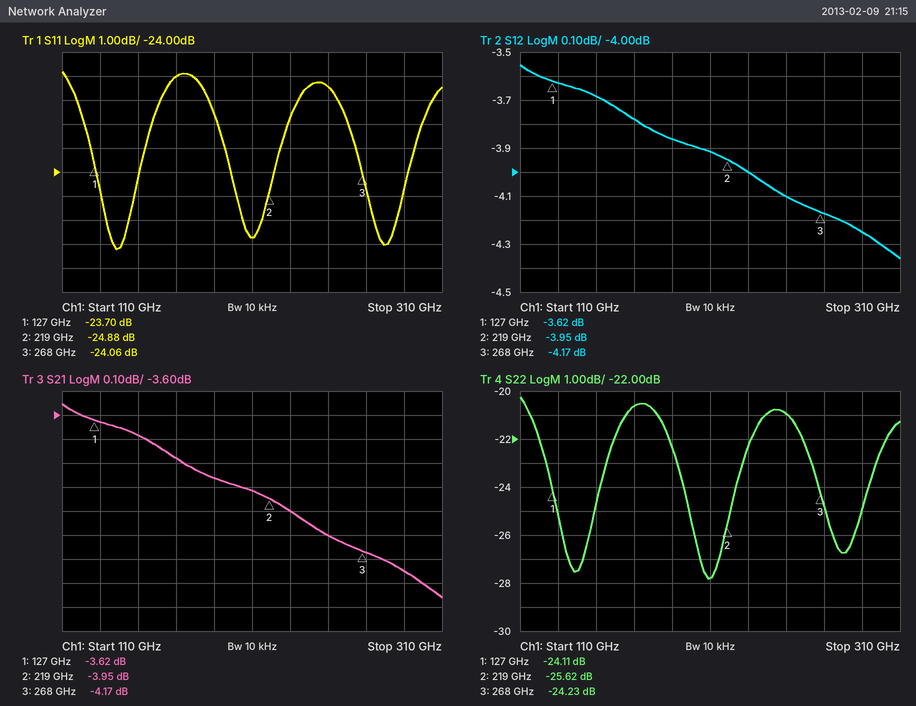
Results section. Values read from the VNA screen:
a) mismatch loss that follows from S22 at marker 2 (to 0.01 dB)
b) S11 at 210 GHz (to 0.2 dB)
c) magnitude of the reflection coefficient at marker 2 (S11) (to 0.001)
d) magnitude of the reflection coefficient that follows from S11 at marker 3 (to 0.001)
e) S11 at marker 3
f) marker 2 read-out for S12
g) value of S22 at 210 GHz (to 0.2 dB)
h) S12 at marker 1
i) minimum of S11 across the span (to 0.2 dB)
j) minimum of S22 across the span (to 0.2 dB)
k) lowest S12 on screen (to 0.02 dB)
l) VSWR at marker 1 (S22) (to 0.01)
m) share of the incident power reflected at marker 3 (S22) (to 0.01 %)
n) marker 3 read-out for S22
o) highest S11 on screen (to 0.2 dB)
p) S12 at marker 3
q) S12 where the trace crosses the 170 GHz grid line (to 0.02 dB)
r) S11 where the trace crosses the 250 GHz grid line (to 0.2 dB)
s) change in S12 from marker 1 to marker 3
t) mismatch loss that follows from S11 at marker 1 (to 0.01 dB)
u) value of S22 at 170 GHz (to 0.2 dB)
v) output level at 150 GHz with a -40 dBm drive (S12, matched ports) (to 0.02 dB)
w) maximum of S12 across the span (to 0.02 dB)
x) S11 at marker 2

0.01 dB
-26.8 dB
0.057
0.063
-24.06 dB
-3.95 dB
-27.8 dB
-3.62 dB
-27.2 dB
-27.8 dB
-4.36 dB
1.13
0.38 %
-24.23 dB
-19.8 dB
-4.17 dB
-3.78 dB
-20.4 dB
-0.55 dB
0.02 dB
-20.6 dB
-43.68 dBm
-3.56 dB
-24.88 dB
